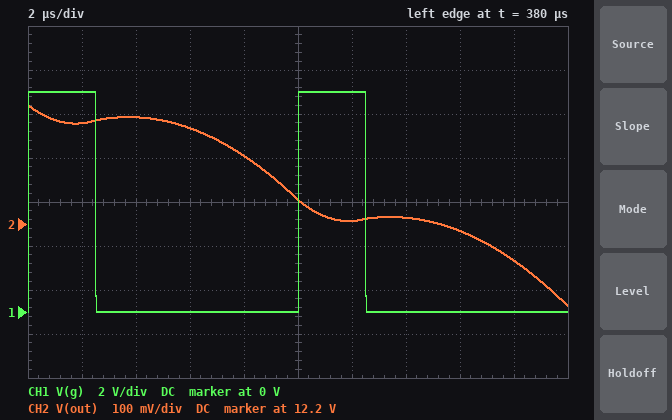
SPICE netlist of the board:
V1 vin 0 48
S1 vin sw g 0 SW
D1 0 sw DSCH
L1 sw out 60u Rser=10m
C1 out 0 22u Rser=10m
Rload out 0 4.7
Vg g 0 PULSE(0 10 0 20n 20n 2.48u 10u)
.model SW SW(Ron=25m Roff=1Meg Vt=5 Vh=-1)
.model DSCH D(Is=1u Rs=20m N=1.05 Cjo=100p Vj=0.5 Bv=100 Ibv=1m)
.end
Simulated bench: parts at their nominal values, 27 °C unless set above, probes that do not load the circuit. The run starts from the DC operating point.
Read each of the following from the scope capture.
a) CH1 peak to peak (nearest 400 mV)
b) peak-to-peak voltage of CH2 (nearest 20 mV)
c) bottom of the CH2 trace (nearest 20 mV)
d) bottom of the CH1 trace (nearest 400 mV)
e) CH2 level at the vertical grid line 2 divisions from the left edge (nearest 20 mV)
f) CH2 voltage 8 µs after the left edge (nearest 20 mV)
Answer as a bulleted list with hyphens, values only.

- 10.0 V
- 460 mV
- 12.02 V
- 0 V
- 12.44 V
- 12.36 V
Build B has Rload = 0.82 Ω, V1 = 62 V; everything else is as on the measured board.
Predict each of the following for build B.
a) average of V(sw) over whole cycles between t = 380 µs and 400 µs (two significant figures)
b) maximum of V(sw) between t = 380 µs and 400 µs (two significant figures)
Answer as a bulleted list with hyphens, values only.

- 15 V
- 62 V
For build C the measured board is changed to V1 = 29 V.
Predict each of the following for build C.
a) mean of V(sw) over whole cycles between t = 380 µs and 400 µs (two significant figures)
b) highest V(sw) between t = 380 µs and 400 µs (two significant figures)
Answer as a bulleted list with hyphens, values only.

- 6.9 V
- 29 V
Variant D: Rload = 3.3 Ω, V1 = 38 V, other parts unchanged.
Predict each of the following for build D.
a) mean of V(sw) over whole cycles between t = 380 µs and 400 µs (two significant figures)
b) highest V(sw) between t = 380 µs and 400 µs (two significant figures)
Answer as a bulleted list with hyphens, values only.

- 9.1 V
- 38 V
